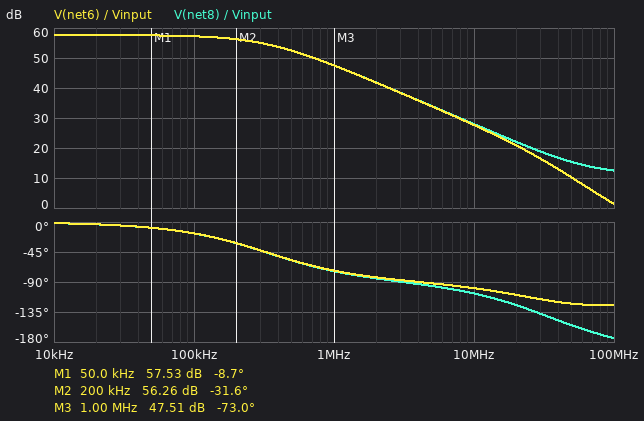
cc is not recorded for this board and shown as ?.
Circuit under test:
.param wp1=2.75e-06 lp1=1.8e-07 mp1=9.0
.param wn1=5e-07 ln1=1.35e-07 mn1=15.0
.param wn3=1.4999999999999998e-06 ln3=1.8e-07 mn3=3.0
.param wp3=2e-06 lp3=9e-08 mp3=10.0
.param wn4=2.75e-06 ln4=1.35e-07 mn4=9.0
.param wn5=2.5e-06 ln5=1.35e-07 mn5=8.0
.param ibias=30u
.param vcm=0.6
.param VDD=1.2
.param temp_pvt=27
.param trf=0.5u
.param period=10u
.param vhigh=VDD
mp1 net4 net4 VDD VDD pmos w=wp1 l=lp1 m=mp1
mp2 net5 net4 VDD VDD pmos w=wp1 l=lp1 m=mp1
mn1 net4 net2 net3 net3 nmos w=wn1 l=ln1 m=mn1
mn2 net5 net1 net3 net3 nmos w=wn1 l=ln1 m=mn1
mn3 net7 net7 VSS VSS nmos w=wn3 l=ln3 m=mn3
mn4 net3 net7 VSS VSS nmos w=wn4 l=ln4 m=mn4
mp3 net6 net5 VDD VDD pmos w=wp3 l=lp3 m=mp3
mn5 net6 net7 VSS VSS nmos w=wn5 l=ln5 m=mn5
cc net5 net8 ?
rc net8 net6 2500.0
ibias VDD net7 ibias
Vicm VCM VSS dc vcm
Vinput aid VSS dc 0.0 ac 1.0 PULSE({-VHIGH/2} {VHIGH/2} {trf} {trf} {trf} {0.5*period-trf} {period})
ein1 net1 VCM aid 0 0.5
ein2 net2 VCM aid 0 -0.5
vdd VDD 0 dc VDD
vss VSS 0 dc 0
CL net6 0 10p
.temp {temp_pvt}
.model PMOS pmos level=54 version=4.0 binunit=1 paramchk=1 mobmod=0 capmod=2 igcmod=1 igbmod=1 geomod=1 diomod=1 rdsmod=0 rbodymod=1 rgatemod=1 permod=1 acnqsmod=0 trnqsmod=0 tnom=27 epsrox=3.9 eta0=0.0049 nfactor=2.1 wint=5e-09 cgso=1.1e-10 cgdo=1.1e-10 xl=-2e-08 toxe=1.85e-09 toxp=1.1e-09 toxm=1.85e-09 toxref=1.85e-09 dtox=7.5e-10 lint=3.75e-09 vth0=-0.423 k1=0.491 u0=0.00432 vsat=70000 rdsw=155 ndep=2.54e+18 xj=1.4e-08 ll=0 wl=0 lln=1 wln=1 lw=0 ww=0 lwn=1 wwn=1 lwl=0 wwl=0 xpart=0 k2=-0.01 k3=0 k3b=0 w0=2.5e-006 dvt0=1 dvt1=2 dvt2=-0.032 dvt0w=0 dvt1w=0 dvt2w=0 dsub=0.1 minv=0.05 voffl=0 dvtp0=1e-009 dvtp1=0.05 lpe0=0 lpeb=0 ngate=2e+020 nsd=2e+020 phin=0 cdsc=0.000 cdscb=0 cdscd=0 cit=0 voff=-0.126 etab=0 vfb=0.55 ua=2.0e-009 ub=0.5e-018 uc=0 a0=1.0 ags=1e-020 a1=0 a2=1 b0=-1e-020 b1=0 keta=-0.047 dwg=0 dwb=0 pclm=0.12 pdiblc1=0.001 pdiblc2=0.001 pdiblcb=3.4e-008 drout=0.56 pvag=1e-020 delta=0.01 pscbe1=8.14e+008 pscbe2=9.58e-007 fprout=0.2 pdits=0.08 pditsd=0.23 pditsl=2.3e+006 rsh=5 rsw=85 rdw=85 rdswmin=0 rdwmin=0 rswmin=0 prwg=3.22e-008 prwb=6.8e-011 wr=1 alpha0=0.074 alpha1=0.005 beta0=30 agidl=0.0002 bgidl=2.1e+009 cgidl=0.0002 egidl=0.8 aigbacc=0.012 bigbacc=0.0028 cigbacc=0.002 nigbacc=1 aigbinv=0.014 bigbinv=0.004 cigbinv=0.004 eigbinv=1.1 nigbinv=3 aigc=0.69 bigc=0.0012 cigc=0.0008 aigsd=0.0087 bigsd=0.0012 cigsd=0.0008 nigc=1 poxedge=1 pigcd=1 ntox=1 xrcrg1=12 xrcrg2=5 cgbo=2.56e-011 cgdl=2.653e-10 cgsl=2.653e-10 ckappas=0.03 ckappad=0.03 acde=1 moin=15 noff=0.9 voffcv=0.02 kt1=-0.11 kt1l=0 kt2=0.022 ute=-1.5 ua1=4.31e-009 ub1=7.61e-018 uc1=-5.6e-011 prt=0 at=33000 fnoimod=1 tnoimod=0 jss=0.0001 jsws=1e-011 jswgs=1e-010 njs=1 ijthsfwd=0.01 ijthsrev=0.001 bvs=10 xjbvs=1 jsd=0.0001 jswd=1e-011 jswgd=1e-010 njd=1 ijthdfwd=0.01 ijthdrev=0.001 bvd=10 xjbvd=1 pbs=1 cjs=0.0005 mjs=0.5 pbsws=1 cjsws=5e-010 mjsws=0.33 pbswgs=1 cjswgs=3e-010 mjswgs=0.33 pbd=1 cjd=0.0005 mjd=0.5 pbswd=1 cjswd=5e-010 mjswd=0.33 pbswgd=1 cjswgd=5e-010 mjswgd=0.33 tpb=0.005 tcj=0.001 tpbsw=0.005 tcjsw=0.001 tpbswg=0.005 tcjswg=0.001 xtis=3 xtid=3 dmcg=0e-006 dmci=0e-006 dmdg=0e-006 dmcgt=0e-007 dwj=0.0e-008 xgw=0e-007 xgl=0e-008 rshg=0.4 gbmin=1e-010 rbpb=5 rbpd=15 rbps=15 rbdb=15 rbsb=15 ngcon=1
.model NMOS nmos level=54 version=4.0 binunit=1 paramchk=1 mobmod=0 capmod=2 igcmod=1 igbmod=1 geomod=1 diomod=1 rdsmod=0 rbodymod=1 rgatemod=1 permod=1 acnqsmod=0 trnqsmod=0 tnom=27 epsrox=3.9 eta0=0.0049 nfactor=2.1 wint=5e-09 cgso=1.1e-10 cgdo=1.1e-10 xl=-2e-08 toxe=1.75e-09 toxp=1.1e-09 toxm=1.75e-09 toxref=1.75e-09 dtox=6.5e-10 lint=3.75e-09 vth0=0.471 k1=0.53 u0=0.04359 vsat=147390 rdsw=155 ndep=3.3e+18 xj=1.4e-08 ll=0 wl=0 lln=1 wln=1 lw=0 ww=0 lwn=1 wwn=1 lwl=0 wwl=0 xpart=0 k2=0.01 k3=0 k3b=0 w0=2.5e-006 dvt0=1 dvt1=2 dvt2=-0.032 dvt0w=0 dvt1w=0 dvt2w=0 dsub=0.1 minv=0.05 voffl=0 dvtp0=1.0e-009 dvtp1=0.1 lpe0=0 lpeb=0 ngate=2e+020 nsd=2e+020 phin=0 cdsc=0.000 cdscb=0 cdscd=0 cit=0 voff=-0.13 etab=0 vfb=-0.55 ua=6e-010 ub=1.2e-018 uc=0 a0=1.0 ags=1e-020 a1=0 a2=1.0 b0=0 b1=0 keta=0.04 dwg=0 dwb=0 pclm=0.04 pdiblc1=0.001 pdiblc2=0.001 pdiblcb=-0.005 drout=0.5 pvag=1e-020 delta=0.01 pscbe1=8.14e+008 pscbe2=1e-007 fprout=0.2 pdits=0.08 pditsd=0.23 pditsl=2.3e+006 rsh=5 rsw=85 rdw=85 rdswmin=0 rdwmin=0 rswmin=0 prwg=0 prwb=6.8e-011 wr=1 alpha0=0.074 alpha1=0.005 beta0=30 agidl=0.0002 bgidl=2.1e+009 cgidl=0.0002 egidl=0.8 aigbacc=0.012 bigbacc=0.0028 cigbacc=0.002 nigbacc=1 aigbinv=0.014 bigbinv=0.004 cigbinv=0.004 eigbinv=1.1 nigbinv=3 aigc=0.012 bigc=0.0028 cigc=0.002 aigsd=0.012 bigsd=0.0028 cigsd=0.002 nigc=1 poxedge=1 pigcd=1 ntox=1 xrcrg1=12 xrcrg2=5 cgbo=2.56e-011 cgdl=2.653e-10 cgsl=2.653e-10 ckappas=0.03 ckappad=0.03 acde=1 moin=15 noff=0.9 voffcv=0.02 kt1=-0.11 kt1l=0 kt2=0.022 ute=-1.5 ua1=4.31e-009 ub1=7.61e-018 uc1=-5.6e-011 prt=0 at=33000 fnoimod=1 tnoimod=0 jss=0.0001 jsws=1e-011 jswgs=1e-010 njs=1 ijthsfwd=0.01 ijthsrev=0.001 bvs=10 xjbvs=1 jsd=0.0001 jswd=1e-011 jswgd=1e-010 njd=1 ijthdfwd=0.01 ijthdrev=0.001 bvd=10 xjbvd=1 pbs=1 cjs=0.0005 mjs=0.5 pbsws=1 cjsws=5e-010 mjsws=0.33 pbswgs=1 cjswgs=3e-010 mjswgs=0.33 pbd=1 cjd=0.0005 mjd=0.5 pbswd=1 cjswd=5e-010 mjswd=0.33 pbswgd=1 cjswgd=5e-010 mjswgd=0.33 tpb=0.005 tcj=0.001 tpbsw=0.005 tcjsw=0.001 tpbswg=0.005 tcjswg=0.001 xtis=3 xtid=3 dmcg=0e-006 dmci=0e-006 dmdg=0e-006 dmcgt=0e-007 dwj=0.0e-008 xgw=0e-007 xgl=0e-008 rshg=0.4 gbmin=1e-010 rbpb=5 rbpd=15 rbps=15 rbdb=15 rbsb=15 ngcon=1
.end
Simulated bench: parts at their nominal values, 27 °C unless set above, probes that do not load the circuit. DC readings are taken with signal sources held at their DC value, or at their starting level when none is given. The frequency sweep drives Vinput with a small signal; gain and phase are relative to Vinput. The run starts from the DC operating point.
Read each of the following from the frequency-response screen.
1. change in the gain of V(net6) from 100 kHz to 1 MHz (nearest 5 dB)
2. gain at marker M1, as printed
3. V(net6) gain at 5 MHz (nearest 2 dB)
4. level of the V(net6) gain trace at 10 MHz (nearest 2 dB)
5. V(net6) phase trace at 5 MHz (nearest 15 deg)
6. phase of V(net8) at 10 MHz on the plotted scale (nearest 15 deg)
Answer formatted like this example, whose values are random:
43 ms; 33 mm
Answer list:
-10 dB; 57.53 dB; 34 dB; 28 dB; -90 deg; -105 deg
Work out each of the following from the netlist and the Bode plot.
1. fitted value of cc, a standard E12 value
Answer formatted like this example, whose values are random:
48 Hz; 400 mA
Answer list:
820 fF
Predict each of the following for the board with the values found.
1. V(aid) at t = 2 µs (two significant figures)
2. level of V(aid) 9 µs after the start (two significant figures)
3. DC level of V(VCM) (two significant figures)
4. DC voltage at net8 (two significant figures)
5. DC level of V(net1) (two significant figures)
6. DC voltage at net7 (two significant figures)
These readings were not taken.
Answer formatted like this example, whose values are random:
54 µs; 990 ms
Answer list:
600 mV; -600 mV; 600 mV; 990 mV; 600 mV; 480 mV
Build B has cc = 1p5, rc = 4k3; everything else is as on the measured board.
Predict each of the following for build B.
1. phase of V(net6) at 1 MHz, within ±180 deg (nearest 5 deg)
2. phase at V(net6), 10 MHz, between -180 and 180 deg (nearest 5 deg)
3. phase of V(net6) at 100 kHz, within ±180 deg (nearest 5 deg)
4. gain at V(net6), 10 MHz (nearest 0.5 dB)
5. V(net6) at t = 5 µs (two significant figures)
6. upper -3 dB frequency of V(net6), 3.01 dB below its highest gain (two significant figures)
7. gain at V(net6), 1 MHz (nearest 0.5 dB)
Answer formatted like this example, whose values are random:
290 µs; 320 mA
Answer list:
-80 deg; -85 deg; -30 deg; 23.5 dB; 1.2 V; 190 kHz; 43.0 dB
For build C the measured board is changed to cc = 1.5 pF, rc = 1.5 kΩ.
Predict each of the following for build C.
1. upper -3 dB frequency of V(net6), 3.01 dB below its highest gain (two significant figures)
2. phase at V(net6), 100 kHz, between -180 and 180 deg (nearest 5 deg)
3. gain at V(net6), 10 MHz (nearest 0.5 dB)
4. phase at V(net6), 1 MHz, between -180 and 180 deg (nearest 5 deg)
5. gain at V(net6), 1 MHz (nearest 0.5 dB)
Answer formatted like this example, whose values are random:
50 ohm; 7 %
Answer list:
190 kHz; -30 deg; 23.0 dB; -80 deg; 43.0 dB
